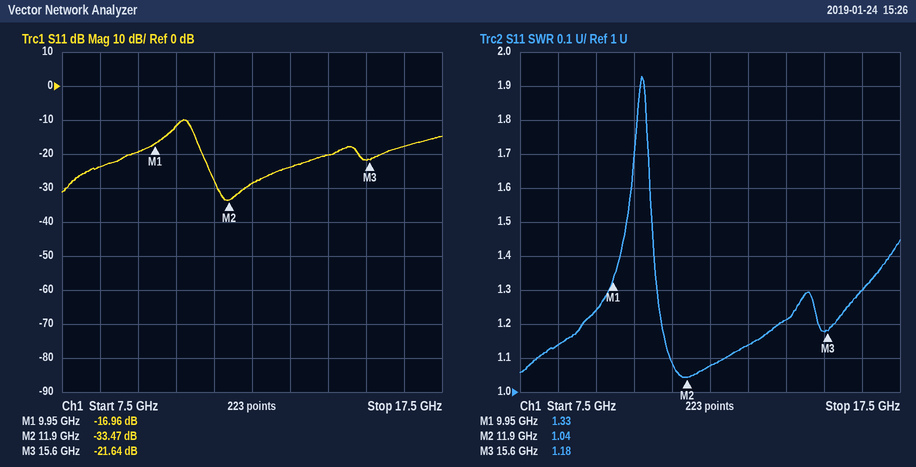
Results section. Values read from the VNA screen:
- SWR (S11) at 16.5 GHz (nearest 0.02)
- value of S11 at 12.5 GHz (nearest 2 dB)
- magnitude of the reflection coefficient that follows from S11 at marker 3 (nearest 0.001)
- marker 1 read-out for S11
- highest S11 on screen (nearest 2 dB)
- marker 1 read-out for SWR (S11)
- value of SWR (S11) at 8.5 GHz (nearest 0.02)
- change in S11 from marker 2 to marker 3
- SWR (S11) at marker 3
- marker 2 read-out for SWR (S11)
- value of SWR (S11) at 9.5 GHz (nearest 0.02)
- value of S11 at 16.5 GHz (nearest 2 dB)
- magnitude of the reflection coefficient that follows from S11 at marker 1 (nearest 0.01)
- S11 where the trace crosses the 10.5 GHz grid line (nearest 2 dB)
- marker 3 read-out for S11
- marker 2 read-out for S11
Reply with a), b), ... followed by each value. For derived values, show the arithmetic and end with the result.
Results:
a) 1.30
b) -28 dB
c) 10^(-21.64/20) ≈ 0.083
d) -16.96 dB
e) -10 dB
f) 1.33
g) 1.14
h) -21.64 − (-33.47) = 11.83 dB
i) 1.18
j) 1.04
k) 1.24
l) -18 dB
m) 10^(-16.96/20) ≈ 0.14
n) -12 dB
o) -21.64 dB
p) -33.47 dB
